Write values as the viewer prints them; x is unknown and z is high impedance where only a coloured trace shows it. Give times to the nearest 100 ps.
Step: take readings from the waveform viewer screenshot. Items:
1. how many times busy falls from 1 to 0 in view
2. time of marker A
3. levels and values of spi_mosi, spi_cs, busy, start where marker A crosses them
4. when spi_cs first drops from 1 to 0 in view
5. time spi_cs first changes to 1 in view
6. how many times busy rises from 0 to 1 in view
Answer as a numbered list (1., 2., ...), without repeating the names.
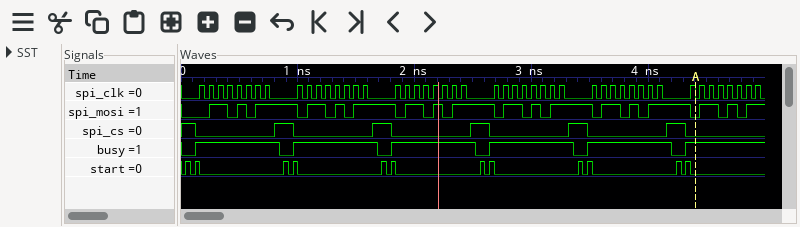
1. 5
2. 4400 ps
3. spi_mosi=0, spi_cs=0, busy=1, start=0
4. 100 ps
5. 800 ps
6. 6
